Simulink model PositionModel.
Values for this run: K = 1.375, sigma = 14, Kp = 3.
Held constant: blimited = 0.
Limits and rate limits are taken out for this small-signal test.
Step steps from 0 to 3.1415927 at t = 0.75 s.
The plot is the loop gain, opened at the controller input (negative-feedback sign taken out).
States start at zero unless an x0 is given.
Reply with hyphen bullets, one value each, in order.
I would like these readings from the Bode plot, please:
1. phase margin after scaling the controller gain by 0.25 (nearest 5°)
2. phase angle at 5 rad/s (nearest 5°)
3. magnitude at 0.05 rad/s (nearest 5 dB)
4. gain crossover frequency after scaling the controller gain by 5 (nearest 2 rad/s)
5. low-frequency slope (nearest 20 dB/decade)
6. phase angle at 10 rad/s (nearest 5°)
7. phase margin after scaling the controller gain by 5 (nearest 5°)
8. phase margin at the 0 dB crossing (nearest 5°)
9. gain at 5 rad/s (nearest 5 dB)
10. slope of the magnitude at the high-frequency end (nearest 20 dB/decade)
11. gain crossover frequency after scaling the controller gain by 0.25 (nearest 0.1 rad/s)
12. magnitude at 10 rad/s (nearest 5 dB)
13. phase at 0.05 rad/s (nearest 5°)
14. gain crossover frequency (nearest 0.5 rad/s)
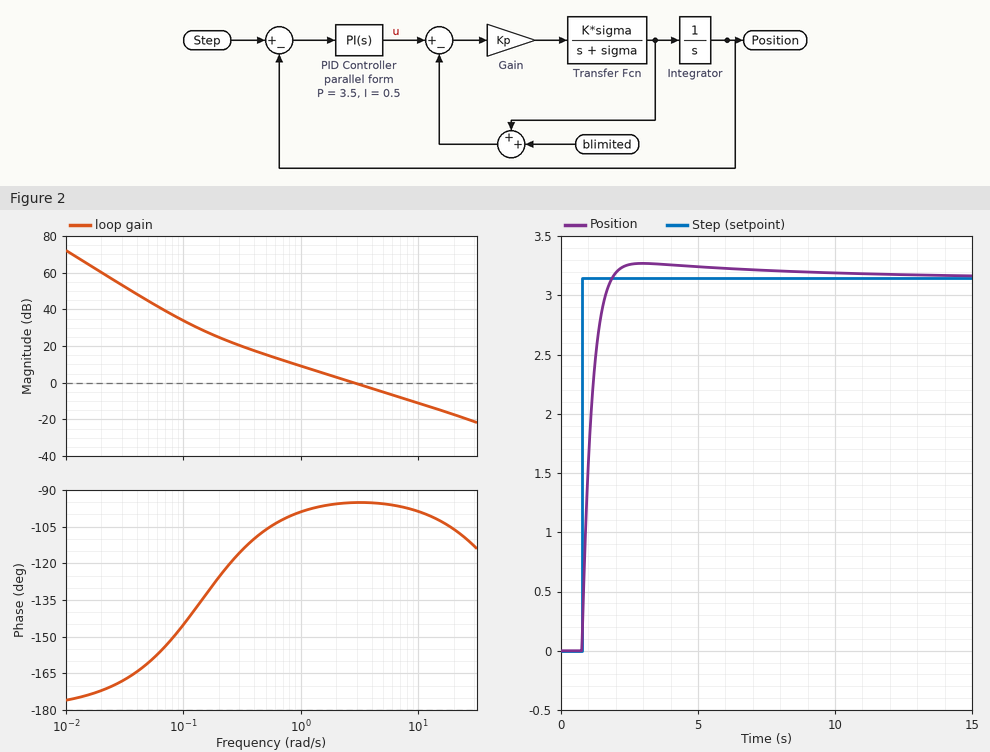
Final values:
- 80°
- -95°
- 45 dB
- 14 rad/s
- -40 dB/decade
- -100°
- 80°
- 85°
- -5 dB
- -20 dB/decade
- 0.7 rad/s
- -10 dB
- -160°
- 3.0 rad/s
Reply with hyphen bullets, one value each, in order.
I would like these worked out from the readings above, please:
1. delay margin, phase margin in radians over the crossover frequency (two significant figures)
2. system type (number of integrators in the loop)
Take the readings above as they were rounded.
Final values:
- 0.49 s
- 2
